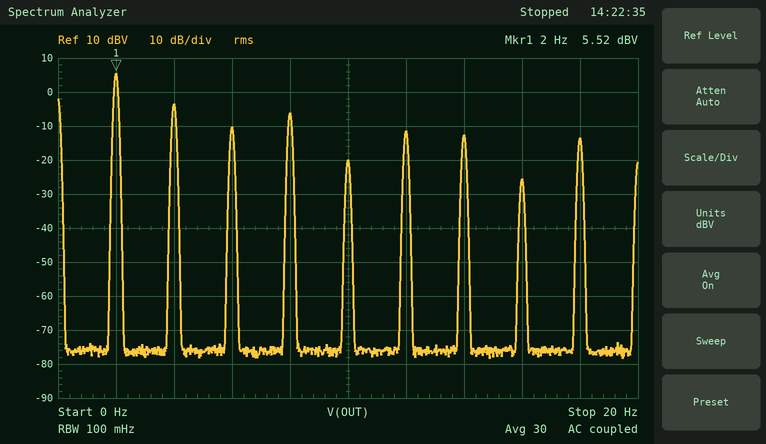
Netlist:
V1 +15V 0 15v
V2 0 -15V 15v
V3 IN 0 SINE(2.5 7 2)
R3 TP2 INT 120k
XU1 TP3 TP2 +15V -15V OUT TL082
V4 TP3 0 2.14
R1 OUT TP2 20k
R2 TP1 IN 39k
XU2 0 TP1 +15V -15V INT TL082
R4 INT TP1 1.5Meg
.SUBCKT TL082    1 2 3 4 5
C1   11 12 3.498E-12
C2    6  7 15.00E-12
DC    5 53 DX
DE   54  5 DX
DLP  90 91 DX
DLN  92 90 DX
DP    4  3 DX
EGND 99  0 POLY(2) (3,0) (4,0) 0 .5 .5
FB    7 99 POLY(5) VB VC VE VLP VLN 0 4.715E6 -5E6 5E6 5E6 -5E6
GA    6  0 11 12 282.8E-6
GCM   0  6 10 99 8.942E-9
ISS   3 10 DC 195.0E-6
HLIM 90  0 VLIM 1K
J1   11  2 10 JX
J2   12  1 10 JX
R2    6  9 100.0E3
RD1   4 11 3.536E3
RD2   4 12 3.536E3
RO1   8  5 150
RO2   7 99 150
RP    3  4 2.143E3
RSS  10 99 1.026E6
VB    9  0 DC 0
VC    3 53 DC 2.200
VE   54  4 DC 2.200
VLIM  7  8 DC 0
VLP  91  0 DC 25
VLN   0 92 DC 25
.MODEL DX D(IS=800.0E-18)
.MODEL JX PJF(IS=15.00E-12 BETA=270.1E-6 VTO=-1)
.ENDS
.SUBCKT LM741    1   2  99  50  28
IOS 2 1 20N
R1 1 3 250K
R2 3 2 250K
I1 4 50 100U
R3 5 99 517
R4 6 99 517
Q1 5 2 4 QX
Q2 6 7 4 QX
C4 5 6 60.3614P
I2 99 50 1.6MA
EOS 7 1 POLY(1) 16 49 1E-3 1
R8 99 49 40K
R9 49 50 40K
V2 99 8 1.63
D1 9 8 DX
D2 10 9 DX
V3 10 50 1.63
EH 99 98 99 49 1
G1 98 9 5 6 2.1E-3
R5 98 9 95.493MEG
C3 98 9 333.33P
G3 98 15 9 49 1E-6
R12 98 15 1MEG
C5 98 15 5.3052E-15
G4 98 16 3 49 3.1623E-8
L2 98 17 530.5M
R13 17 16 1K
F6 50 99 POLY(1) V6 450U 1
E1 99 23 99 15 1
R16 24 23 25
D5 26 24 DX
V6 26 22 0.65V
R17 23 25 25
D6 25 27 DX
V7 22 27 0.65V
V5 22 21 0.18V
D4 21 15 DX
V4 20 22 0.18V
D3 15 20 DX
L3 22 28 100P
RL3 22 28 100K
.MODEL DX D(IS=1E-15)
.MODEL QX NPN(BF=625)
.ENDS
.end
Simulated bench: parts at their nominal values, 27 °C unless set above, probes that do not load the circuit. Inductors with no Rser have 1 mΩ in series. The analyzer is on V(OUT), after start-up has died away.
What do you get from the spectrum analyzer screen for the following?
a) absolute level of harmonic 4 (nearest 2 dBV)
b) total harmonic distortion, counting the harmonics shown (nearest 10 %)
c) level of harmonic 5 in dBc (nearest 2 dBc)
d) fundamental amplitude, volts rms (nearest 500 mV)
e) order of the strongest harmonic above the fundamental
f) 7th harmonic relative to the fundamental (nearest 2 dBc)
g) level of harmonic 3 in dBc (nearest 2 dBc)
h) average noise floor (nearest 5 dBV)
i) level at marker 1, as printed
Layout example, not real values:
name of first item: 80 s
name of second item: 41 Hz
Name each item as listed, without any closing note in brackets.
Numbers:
absolute level of harmonic 4: -6 dBV
total harmonic distortion, counting the harmonics shown: 50 %
level of harmonic 5 in dBc: -26 dBc
fundamental amplitude, volts rms: 2.0 V
order of the strongest harmonic above the fundamental: 2
7th harmonic relative to the fundamental: -18 dBc
level of harmonic 3 in dBc: -16 dBc
average noise floor: -75 dBV
level at marker 1, as printed: 5.52 dBV
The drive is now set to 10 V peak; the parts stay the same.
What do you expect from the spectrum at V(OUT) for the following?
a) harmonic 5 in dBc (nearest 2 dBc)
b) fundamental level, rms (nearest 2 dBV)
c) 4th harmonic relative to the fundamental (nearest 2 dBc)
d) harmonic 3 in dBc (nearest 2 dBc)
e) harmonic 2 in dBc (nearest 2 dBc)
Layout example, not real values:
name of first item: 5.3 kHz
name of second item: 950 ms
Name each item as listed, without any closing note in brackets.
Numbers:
harmonic 5 in dBc: -24 dBc
fundamental level, rms: 6 dBV
4th harmonic relative to the fundamental: -14 dBc
harmonic 3 in dBc: -12 dBc
harmonic 2 in dBc: -12 dBc
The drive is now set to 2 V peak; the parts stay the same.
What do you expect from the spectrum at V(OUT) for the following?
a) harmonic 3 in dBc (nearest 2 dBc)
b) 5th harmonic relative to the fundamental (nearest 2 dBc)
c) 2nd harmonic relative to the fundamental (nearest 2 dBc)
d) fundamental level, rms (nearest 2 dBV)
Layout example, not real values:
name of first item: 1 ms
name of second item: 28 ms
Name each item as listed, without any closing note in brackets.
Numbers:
harmonic 3 in dBc: -4 dBc
5th harmonic relative to the fundamental: -12 dBc
2nd harmonic relative to the fundamental: -2 dBc
fundamental level, rms: -60 dBV
